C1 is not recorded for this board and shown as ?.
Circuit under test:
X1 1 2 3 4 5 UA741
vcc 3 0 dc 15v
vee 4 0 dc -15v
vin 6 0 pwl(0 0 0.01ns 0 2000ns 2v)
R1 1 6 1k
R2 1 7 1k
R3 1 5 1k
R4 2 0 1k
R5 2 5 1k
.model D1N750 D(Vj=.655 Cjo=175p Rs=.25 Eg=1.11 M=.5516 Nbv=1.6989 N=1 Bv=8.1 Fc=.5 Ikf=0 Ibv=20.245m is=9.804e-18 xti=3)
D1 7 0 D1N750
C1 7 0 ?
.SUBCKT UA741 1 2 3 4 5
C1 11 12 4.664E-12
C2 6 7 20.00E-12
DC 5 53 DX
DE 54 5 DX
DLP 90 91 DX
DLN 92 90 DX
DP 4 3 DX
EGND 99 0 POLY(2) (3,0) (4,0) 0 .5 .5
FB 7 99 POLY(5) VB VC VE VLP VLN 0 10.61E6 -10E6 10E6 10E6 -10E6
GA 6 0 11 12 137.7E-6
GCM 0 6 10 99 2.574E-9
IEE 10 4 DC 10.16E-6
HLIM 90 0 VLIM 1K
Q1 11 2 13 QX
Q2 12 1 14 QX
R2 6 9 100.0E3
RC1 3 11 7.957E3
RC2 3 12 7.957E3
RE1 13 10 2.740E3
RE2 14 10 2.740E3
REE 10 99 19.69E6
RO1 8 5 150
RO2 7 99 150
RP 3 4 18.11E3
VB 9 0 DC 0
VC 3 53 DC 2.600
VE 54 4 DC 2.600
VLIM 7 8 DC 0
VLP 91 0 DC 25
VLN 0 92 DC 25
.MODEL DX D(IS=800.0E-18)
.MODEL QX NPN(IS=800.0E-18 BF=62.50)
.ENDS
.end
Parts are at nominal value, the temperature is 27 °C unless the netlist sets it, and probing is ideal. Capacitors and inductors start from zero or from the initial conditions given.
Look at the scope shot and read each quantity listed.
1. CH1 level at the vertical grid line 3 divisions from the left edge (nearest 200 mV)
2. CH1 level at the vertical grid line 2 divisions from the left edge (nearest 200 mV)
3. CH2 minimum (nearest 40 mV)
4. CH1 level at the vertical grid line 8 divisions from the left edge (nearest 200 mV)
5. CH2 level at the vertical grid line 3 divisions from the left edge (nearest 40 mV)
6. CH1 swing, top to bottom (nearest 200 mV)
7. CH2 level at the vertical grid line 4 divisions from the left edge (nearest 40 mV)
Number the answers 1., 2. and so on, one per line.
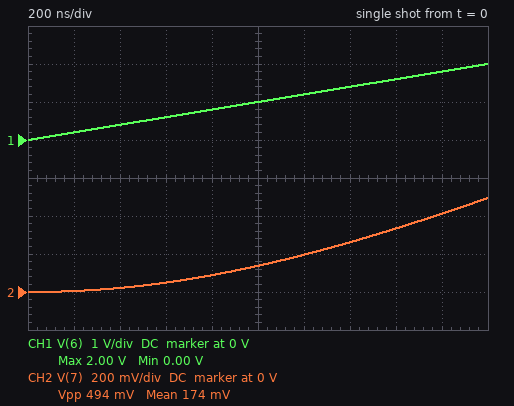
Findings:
1. 600 mV
2. 400 mV
3. 0 V
4. 1.6 V
5. 40 mV
6. 2.0 V
7. 80 mV
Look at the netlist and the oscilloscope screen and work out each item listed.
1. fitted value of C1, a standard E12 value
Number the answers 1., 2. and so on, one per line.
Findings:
1. 1.2 nF
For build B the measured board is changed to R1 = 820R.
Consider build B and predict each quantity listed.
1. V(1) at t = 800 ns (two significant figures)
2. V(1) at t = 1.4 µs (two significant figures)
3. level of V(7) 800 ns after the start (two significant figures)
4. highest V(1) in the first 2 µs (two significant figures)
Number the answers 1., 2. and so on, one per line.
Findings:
1. 430 mV
2. 810 mV
3. 97 mV
4. 1.2 V
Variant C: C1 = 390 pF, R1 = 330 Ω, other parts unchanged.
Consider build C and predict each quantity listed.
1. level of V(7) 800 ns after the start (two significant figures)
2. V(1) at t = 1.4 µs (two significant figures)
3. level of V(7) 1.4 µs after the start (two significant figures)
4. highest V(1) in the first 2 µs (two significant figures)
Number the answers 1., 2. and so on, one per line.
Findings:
1. 260 mV
2. 1.1 V
3. 620 mV
4. 1.6 V
